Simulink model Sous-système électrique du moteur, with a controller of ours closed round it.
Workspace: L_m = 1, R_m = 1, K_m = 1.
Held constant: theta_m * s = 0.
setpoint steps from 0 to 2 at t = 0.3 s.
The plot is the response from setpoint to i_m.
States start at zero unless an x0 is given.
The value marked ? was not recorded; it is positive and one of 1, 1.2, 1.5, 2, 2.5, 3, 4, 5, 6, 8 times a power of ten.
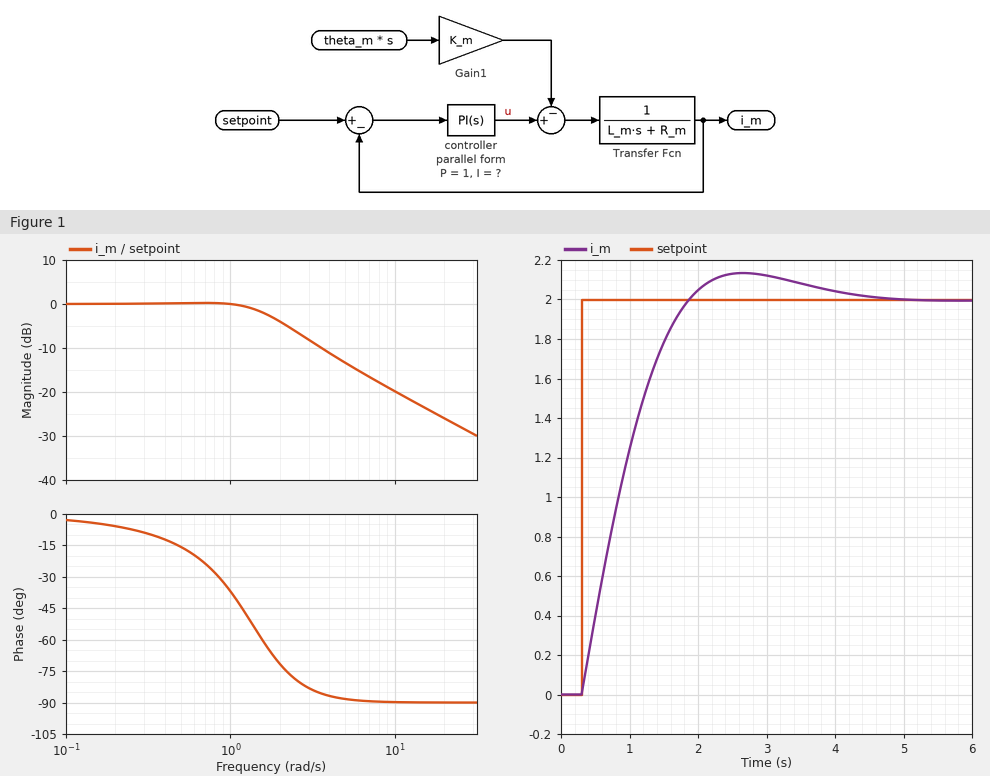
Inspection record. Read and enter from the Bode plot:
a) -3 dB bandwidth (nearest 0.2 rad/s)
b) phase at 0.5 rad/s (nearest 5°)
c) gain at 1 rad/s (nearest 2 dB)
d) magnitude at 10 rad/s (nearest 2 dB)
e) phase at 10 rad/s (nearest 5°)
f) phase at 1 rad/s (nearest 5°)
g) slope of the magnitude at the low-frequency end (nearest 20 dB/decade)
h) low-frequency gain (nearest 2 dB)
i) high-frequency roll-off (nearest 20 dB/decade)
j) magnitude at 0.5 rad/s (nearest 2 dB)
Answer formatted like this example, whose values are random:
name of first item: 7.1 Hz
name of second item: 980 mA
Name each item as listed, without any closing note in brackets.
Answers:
-3 dB bandwidth: 1.8 rad/s
phase at 0.5 rad/s: -15°
gain at 1 rad/s: 0 dB
magnitude at 10 rad/s: -20 dB
phase at 10 rad/s: -90°
phase at 1 rad/s: -35°
slope of the magnitude at the low-frequency end: 0 dB/decade
low-frequency gain: 0 dB
high-frequency roll-off: -20 dB/decade
magnitude at 0.5 rad/s: 0 dB
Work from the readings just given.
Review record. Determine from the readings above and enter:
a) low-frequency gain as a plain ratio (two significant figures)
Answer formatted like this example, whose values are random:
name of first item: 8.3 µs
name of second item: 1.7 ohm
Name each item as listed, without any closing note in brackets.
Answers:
low-frequency gain as a plain ratio: 1.0
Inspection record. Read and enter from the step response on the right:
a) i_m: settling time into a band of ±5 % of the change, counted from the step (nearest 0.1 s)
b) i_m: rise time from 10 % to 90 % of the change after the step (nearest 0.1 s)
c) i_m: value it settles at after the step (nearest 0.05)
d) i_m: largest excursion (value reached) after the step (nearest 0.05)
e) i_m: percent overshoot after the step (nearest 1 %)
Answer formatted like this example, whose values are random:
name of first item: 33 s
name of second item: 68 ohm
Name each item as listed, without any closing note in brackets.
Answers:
i_m: settling time into a band of ±5 % of the change, counted from the step: 3.0 s
i_m: rise time from 10 % to 90 % of the change after the step: 1.1 s
i_m: value it settles at after the step: 2.00
i_m: largest excursion (value reached) after the step: 2.15
i_m: percent overshoot after the step: 7 %
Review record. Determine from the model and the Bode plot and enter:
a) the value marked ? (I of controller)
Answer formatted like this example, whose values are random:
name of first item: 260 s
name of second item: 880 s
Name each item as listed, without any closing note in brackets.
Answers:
the value marked ?: 2
